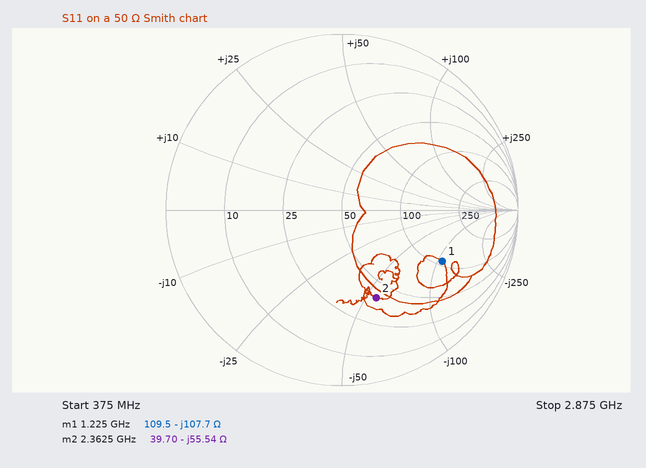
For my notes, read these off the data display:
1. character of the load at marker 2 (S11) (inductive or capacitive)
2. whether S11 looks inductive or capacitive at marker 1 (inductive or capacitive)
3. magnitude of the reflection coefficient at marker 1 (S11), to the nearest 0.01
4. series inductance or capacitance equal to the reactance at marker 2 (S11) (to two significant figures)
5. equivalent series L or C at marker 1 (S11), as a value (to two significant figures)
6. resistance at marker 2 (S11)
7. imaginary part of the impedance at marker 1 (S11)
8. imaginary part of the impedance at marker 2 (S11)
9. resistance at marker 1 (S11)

capacitive
capacitive
0.64
1.2 pF
1.2 pF
39.70 Ω
-107.7 Ω
-55.54 Ω
109.5 Ω
